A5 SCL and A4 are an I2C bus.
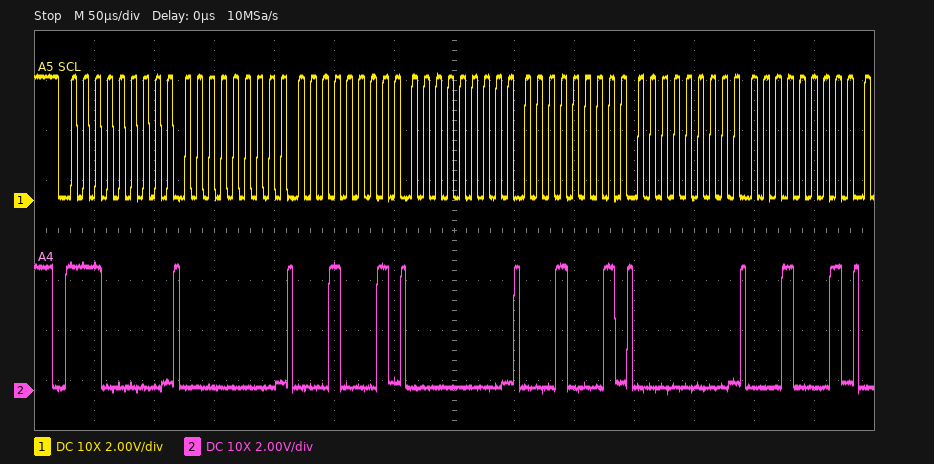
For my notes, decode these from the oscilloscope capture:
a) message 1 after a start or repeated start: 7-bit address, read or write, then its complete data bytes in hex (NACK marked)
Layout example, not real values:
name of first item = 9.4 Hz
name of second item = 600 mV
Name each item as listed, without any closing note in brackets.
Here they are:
message 1 after a start or repeated start: 7-bit address, read or write, then its complete data bytes in hex = 0x70 write: 00 11 00 11 00 11
